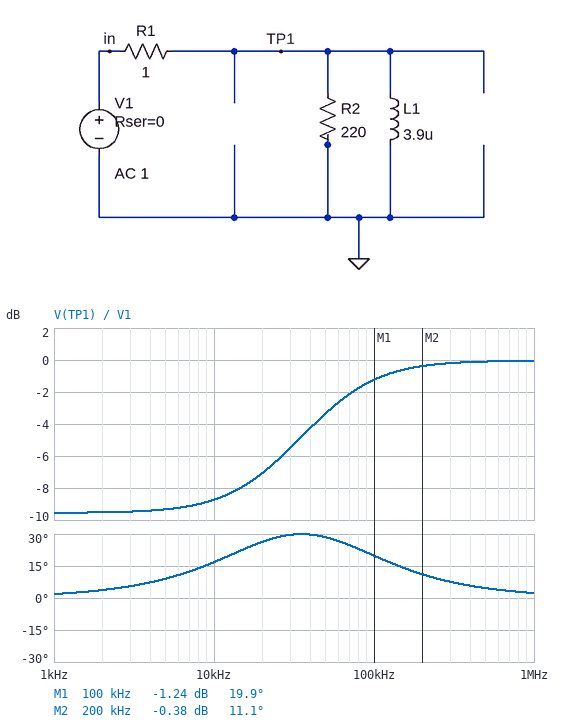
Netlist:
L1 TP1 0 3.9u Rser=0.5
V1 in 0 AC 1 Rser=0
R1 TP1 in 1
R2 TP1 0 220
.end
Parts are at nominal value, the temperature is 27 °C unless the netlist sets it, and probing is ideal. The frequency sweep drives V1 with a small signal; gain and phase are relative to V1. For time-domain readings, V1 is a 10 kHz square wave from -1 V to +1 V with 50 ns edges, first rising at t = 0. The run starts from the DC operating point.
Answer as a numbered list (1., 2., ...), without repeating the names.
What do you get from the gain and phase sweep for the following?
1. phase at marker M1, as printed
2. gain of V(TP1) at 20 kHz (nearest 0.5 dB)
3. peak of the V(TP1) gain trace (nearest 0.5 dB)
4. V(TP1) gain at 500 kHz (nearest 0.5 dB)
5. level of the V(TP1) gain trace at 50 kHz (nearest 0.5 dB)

1. 19.9 deg
2. -7.0 dB
3. 0 dB
4. 0 dB
5. -3.5 dB
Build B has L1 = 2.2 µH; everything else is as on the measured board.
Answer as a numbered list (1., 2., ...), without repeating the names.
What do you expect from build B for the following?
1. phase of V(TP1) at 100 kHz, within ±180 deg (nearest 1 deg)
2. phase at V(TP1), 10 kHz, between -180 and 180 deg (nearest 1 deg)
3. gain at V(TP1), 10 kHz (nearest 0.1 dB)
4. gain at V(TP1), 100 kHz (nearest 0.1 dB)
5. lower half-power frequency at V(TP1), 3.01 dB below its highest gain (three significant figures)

1. 27 deg
2. 10 deg
3. -9.3 dB
4. -2.9 dB
5. 95.3 kHz
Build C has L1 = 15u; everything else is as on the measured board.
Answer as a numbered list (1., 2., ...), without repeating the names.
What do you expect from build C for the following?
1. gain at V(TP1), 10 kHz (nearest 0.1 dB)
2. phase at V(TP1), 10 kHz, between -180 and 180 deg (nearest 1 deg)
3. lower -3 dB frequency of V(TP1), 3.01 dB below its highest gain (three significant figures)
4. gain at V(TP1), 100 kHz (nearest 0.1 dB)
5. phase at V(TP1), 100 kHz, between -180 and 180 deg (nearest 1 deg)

1. -4.4 dB
2. 30 deg
3. 14.0 kHz
4. -0.1 dB
5. 6 deg
